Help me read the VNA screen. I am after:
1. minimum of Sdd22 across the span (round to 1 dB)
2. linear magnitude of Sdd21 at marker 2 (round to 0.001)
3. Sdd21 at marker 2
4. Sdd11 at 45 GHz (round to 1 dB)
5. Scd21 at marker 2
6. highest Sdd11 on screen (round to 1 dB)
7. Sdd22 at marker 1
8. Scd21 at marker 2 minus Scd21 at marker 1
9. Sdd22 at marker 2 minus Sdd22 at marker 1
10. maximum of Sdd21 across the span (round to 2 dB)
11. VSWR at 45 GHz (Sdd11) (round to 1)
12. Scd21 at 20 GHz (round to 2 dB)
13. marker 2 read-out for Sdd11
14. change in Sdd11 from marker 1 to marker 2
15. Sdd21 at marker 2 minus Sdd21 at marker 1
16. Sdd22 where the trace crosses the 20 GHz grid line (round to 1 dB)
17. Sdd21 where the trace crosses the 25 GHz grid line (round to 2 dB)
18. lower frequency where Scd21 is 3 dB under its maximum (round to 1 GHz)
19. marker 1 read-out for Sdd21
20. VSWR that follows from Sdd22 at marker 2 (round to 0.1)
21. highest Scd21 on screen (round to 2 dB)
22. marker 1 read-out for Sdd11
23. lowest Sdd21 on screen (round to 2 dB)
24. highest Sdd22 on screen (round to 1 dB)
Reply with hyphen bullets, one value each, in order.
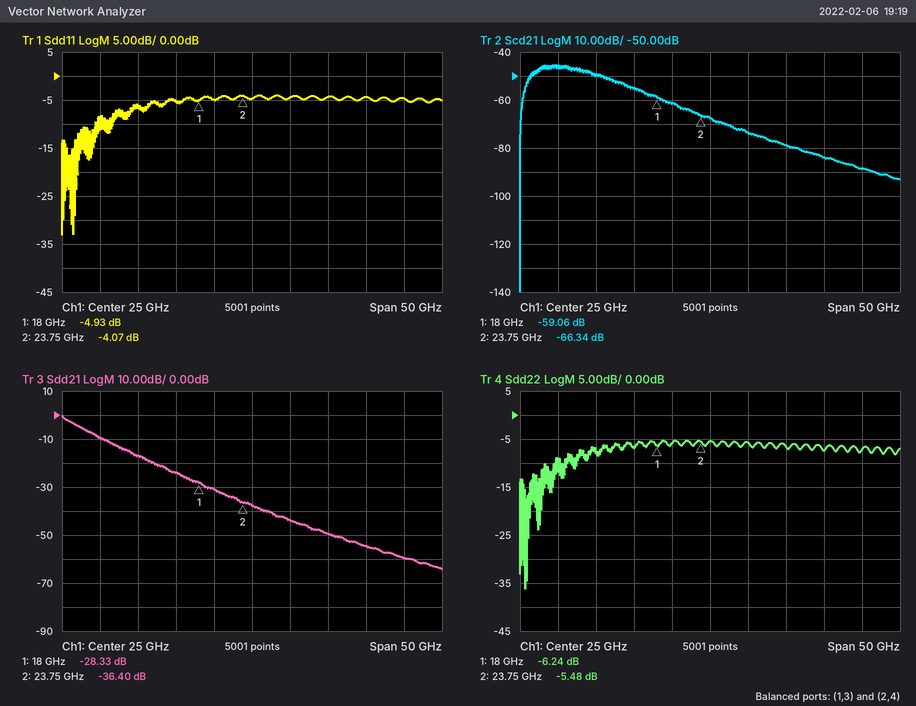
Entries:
- -36 dB
- 0.015
- -36.40 dB
- -5 dB
- -66.34 dB
- -4 dB
- -6.24 dB
- -7.28 dB
- 0.76 dB
- 0 dB
- 4
- -62 dB
- -4.07 dB
- 0.86 dB
- -8.07 dB
- -6 dB
- -38 dB
- 2 GHz
- -28.33 dB
- 3.3
- -46 dB
- -4.93 dB
- -64 dB
- -5 dB
